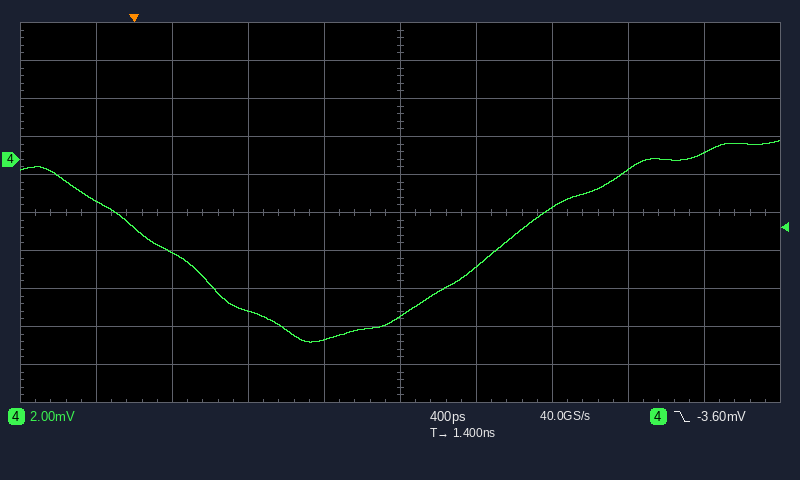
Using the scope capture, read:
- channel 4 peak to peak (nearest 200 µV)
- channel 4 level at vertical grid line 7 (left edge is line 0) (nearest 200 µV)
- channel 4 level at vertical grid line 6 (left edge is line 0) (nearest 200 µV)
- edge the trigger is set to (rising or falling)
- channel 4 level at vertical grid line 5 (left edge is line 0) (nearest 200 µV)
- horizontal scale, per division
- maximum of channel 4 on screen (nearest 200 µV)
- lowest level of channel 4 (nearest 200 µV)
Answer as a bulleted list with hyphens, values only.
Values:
- 10.6 mV
- -2.6 mV
- -5.6 mV
- falling
- -8.2 mV
- 400 ps
- 1.0 mV
- -9.6 mV
